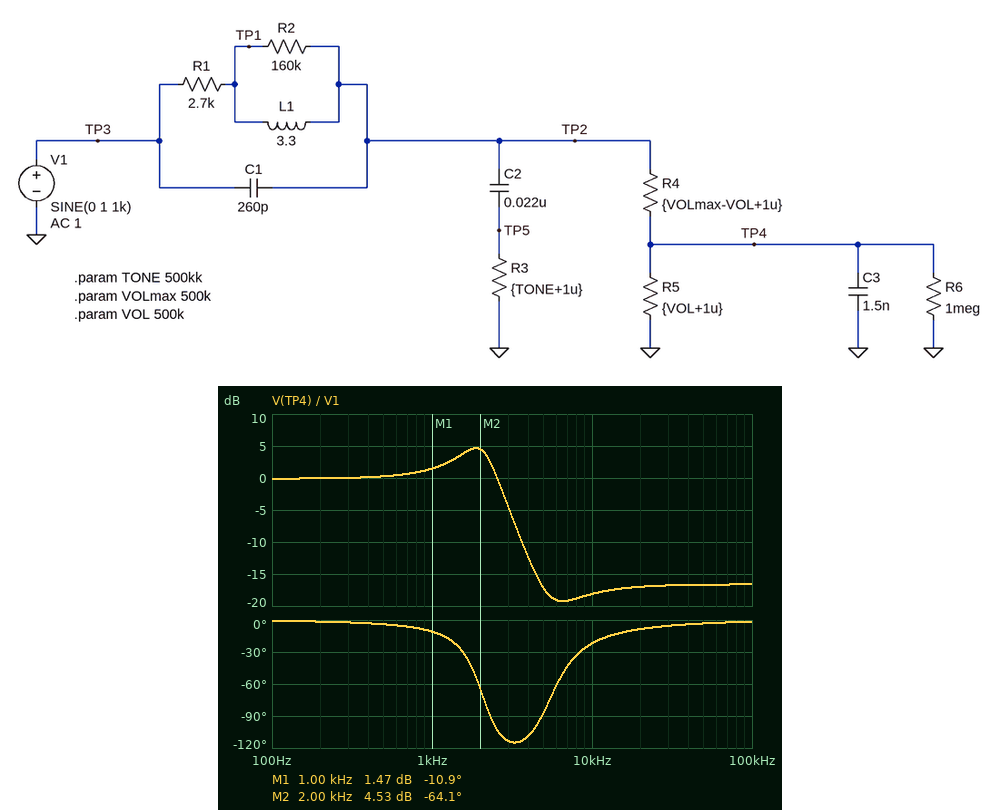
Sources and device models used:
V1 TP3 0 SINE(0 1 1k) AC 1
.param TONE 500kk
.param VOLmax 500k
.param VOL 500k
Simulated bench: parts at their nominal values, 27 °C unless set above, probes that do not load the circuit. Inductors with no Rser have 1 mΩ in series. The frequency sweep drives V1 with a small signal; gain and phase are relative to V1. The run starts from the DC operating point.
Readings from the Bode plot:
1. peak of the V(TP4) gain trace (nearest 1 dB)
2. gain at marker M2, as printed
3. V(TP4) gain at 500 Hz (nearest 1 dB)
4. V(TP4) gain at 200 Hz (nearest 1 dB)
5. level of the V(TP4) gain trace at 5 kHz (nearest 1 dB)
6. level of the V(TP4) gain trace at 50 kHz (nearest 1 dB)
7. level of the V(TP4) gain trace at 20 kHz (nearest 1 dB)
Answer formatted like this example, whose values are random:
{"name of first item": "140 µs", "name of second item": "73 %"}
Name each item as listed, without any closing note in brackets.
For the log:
{"peak of the V(TP4) gain trace": "5 dB", "gain at marker M2, as printed": "4.53 dB", "V(TP4) gain at 500 Hz": "0 dB", "V(TP4) gain at 200 Hz": "0 dB", "level of the V(TP4) gain trace at 5 kHz": "-17 dB", "level of the V(TP4) gain trace at 50 kHz": "-17 dB", "level of the V(TP4) gain trace at 20 kHz": "-17 dB"}
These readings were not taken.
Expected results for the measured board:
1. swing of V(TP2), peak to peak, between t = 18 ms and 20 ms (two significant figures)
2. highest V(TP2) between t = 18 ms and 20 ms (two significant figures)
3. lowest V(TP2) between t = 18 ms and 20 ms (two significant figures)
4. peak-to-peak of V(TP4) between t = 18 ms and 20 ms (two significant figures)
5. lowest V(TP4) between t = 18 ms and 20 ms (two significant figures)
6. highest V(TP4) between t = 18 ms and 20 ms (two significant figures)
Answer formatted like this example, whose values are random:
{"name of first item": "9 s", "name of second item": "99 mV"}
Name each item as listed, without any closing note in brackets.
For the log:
{"swing of V(TP2), peak to peak, between t = 18 ms and 20 ms": "2.4 V", "highest V(TP2) between t = 18 ms and 20 ms": "1.2 V", "lowest V(TP2) between t = 18 ms and 20 ms": "-1.2 V", "peak-to-peak of V(TP4) between t = 18 ms and 20 ms": "2.4 V", "lowest V(TP4) between t = 18 ms and 20 ms": "-1.2 V", "highest V(TP4) between t = 18 ms and 20 ms": "1.2 V"}
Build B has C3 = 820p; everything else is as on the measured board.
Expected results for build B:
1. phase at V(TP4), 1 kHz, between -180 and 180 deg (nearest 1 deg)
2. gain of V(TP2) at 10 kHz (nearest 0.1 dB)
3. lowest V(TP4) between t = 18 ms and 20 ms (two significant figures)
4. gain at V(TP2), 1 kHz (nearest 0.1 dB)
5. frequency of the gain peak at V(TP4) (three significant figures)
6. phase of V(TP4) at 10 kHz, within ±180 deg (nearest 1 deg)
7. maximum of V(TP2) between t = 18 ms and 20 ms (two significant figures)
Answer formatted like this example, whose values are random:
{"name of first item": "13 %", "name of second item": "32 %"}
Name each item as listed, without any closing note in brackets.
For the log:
{"phase at V(TP4), 1 kHz, between -180 and 180 deg": "-8 deg", "gain of V(TP2) at 10 kHz": "-13.7 dB", "lowest V(TP4) between t = 18 ms and 20 ms": "-1.1 V", "gain at V(TP2), 1 kHz": "0.6 dB", "frequency of the gain peak at V(TP4)": "2.24 kHz", "phase of V(TP4) at 10 kHz, within ±180 deg": "-18 deg", "maximum of V(TP2) between t = 18 ms and 20 ms": "1.1 V"}
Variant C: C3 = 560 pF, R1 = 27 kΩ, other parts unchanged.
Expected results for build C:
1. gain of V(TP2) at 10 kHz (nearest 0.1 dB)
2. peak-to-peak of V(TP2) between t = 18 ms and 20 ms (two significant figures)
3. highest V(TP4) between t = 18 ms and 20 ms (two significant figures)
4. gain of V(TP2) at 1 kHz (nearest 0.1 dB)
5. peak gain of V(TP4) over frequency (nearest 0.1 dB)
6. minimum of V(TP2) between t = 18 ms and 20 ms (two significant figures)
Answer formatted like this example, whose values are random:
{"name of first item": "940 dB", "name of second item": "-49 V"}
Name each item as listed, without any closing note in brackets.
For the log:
{"gain of V(TP2) at 10 kHz": "-10.9 dB", "peak-to-peak of V(TP2) between t = 18 ms and 20 ms": "1.8 V", "highest V(TP4) between t = 18 ms and 20 ms": "900 mV", "gain of V(TP2) at 1 kHz": "-0.9 dB", "peak gain of V(TP4) over frequency": "-0.7 dB", "minimum of V(TP2) between t = 18 ms and 20 ms": "-900 mV"}
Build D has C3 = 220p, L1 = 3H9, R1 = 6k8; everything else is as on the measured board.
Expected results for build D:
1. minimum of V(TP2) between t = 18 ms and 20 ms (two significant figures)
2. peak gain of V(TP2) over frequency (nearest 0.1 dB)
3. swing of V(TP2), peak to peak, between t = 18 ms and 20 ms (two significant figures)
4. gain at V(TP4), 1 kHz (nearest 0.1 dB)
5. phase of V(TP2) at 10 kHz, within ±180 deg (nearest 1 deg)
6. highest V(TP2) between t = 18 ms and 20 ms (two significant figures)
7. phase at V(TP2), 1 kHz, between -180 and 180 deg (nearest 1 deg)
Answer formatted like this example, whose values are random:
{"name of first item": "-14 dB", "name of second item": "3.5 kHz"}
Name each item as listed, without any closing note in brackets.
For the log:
{"minimum of V(TP2) between t = 18 ms and 20 ms": "-970 mV", "peak gain of V(TP2) over frequency": "-0.2 dB", "swing of V(TP2), peak to peak, between t = 18 ms and 20 ms": "1.9 V", "gain at V(TP4), 1 kHz": "-0.3 dB", "phase of V(TP2) at 10 kHz, within ±180 deg": "-3 deg", "highest V(TP2) between t = 18 ms and 20 ms": "970 mV", "phase at V(TP2), 1 kHz, between -180 and 180 deg": "-8 deg"}
